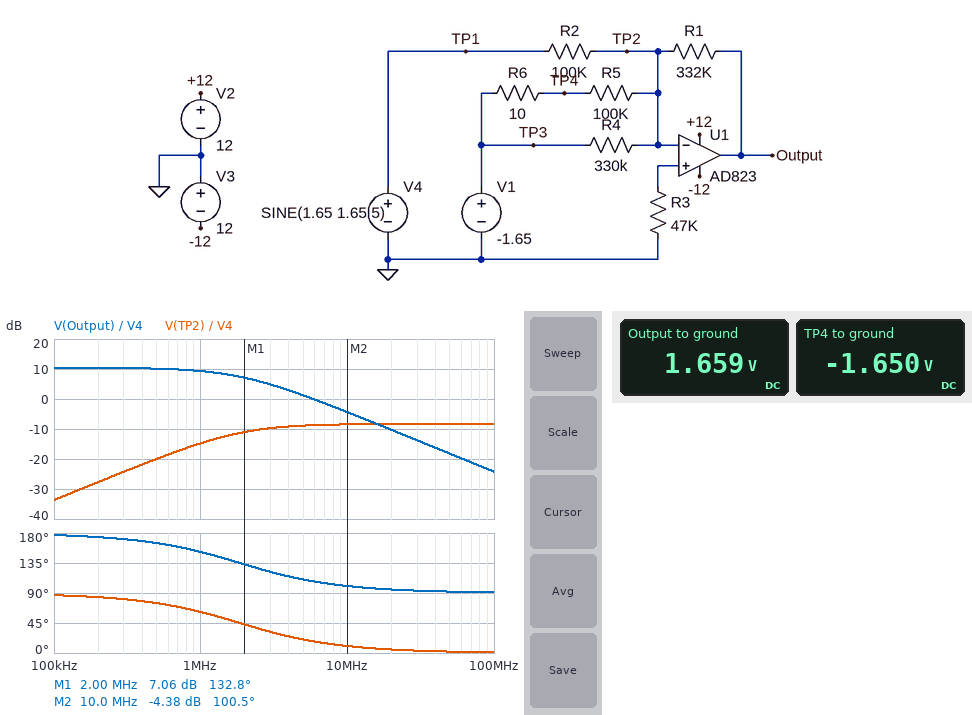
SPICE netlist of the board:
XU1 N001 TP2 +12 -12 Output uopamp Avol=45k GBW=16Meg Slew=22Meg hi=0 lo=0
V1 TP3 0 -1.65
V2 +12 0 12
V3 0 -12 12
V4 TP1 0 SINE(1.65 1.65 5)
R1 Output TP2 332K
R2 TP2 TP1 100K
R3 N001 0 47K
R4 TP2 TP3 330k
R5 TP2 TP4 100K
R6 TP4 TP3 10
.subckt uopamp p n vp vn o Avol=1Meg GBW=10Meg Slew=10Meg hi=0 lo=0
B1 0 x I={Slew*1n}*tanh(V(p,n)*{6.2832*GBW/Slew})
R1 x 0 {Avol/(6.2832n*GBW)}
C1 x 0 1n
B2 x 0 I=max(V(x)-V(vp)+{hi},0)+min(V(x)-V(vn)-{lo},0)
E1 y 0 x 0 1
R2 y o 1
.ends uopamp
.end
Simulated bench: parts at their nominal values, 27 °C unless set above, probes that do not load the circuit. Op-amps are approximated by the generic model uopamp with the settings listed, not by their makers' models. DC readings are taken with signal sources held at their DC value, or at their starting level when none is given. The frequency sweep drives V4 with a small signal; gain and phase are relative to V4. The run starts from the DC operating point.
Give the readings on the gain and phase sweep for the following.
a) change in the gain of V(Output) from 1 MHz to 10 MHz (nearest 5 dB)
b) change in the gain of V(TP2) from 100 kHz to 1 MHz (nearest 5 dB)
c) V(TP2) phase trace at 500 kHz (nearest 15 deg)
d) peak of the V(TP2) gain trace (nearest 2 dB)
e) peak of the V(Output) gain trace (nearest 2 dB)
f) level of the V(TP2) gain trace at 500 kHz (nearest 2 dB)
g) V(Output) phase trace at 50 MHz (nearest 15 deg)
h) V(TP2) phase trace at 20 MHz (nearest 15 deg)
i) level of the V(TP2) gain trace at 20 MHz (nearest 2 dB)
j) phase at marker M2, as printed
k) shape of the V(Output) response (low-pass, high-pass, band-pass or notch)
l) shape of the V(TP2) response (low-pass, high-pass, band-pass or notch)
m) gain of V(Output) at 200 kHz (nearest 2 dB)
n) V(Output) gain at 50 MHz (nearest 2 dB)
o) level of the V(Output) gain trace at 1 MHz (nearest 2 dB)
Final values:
-15 dB
20 dB
75 deg
-8 dB
10 dB
-20 dB
90 deg
0 deg
-8 dB
100.5 deg
low-pass
high-pass
10 dB
-18 dB
10 dB
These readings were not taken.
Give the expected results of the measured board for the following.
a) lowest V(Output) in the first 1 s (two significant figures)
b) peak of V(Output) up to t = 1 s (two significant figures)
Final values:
-3.8 V
7.1 V
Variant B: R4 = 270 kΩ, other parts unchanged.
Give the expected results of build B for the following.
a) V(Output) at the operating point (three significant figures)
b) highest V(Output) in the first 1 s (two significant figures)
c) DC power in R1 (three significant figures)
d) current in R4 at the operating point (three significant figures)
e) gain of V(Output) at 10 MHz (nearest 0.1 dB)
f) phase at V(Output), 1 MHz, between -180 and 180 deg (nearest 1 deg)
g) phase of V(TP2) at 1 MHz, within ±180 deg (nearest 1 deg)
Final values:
2.03 V
7.5 V
12.4 µW
6.11 µA
-4.6 dB
151 deg
61 deg
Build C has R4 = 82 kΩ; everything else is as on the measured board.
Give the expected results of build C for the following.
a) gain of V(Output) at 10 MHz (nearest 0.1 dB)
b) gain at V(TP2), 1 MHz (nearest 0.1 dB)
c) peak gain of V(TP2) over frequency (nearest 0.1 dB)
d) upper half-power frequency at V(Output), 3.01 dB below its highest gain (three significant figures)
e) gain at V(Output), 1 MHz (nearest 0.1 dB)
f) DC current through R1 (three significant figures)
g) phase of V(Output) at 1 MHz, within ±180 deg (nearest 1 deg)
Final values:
-6.9 dB
-15.5 dB
-10.9 dB
1.37 MHz
8.6 dB
20.1 µA
144 deg
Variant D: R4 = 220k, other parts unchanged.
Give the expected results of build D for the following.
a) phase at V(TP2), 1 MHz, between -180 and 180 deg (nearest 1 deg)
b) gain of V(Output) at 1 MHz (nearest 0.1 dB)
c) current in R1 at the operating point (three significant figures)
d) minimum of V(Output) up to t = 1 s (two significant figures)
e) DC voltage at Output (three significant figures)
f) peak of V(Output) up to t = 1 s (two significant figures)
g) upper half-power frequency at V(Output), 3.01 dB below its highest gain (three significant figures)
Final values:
60 deg
9.2 dB
7.50 µA
-3.0 V
2.49 V
8.0 V
1.75 MHz
